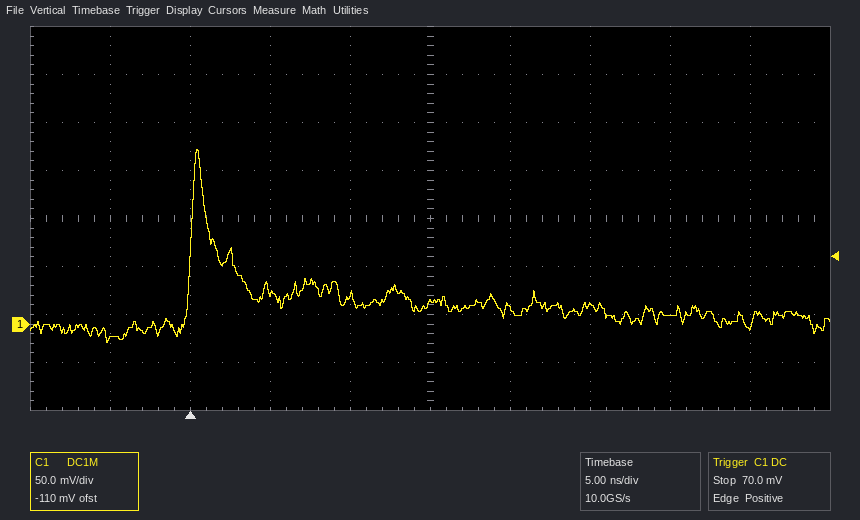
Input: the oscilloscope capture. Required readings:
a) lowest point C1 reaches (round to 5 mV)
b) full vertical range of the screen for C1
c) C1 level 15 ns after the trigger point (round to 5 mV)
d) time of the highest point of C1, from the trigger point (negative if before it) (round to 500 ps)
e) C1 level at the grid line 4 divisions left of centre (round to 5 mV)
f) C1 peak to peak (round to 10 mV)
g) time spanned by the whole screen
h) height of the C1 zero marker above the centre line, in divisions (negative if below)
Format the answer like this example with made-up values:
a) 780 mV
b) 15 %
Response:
a) -20 mV
b) 400 mV
c) 20 mV
d) +500 ps
e) -15 mV
f) 200 mV
g) 50 ns
h) -2.2 div
